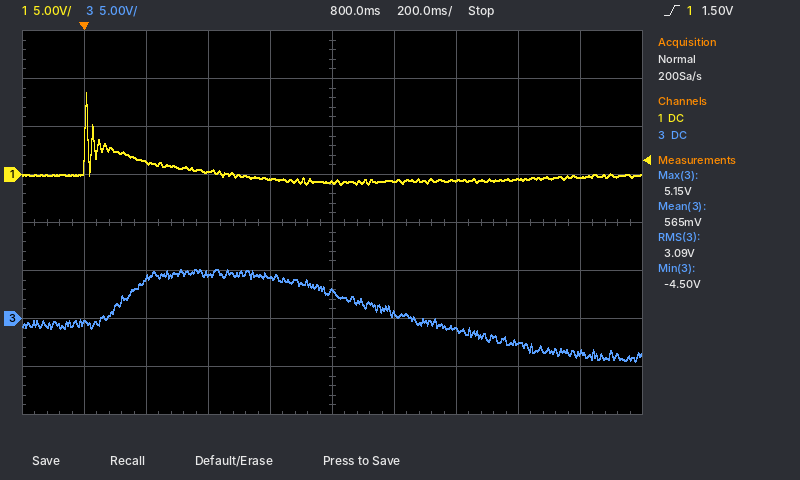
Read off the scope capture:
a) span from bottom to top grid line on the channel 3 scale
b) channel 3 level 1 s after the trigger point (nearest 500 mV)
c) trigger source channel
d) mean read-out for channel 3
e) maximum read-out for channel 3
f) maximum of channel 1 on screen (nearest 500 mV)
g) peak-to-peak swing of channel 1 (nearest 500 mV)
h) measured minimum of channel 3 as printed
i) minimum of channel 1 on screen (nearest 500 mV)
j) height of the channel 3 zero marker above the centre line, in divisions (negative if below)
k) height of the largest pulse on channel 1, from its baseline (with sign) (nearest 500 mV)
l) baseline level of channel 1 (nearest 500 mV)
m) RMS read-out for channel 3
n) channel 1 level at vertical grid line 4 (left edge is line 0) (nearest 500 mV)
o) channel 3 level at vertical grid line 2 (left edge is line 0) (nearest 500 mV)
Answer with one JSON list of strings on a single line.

["40 V", "500 mV", "channel 1", "565 mV", "5.15 V", "8.5 V", "9.5 V", "-4.50 V", "-1.0 V", "-2.0 div", "+9.0 V", "-500 mV", "3.09 V", "-500 mV", "4.0 V"]
